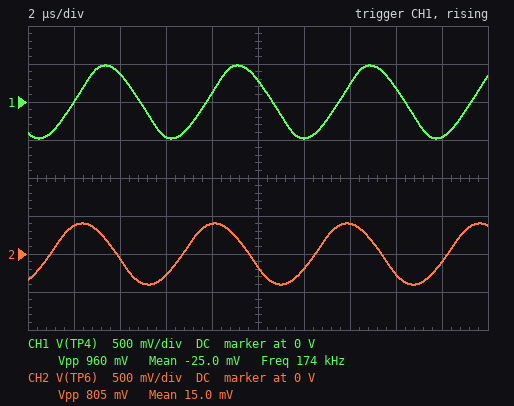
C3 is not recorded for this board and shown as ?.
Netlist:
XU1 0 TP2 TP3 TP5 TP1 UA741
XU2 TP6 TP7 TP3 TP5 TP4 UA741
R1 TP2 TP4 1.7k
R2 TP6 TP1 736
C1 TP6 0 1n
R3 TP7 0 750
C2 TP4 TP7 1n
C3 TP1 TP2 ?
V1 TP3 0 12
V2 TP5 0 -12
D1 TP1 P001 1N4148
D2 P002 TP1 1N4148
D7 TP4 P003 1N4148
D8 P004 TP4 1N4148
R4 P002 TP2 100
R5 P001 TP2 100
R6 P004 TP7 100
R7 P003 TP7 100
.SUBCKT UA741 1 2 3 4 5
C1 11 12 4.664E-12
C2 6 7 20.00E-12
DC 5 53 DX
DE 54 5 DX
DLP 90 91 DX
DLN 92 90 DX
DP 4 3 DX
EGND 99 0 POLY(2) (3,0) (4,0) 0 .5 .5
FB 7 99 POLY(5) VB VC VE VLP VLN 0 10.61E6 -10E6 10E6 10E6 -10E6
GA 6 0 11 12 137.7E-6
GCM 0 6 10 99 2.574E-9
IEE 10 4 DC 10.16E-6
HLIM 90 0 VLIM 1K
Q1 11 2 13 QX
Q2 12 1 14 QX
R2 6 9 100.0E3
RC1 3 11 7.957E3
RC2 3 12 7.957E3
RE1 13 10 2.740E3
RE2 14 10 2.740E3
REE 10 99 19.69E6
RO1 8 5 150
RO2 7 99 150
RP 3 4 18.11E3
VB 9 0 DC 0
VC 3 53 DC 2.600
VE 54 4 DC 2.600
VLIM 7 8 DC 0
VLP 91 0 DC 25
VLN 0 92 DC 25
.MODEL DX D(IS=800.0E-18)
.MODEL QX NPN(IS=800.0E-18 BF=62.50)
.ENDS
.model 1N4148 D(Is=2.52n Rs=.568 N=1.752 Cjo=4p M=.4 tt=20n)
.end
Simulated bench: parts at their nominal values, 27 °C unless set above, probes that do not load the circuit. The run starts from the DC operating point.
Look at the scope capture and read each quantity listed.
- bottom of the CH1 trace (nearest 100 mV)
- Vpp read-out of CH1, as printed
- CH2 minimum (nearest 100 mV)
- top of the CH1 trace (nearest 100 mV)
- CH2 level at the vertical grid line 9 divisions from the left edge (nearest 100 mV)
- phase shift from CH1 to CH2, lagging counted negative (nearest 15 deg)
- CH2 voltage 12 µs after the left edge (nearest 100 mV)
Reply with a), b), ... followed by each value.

a) -500 mV
b) 960 mV
c) -400 mV
d) 500 mV
e) -100 mV
f) 60 deg
g) -200 mV
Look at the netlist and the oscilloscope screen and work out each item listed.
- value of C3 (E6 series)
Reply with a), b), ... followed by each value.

a) 68 pF
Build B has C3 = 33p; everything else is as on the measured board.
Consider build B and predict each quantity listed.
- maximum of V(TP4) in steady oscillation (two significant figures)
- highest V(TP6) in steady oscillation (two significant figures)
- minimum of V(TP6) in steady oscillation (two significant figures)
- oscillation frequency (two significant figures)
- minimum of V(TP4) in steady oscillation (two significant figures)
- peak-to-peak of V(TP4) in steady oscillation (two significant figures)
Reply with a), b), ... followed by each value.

a) 460 mV
b) 390 mV
c) -390 mV
d) 180 kHz
e) -460 mV
f) 920 mV
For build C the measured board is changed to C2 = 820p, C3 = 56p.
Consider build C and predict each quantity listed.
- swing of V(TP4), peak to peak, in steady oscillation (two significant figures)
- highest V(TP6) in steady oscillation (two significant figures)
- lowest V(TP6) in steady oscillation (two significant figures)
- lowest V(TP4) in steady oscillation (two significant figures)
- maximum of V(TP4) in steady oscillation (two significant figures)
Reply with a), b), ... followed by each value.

a) 1.1 V
b) 420 mV
c) -420 mV
d) -550 mV
e) 550 mV
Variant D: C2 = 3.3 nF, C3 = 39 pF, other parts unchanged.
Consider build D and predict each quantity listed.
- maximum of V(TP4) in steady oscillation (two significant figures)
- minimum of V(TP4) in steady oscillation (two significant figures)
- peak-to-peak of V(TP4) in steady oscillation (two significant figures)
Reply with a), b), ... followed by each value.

a) 250 mV
b) -250 mV
c) 510 mV
